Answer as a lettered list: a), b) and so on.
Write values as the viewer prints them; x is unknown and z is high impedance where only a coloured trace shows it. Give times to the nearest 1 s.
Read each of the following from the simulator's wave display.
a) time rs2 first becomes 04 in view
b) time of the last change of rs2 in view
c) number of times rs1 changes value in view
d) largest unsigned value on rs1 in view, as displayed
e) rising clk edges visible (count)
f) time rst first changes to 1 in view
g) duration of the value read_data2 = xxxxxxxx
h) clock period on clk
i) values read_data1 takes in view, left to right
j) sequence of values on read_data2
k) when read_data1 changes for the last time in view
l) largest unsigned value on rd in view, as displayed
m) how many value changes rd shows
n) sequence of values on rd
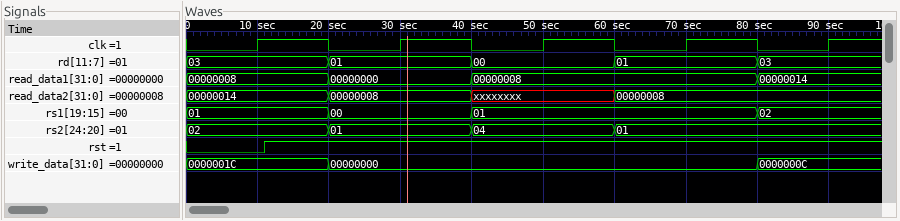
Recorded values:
a) 40 s
b) 60 s
c) 3
d) 02
e) 5
f) 11 s
g) 20 s
h) 20 s
i) 00000008, 00000000, 00000008, 00000014
j) 00000014, 00000008, xxxxxxxx, 00000008
k) 80 s
l) 03
m) 4
n) 03, 01, 00, 01, 03
